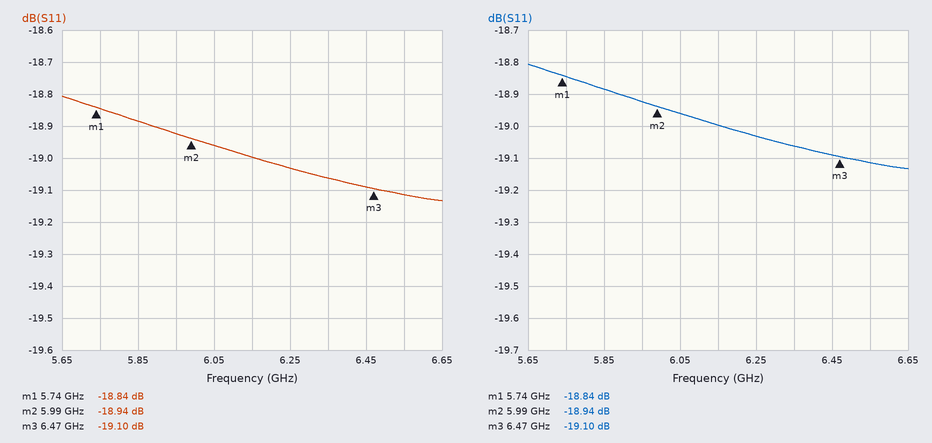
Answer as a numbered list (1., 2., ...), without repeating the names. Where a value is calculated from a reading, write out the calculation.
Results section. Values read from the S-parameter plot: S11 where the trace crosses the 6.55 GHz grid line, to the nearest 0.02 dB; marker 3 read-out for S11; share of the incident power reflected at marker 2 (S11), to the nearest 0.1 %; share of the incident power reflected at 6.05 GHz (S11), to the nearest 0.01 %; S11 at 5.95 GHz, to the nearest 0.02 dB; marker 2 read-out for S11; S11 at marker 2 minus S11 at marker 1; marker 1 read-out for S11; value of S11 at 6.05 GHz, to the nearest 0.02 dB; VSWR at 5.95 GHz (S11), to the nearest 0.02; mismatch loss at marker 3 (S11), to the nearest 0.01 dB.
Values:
1. -19.12 dB
2. -19.10 dB
3. 10^(-18.94/10) ≈ 1.3 %
4. 10^(-18.96/10) ≈ 1.27 %
5. -18.92 dB
6. -18.94 dB
7. -18.94 − (-18.84) = -0.10 dB
8. -18.84 dB
9. -18.96 dB
10. |Γ| = 10^(-18.92/20) = 0.1132; VSWR = (1 + 0.1132)/(1 − 0.1132) ≈ 1.26
11. −10 log10(1 − 10^(-19.1/10)) ≈ 0.05 dB
